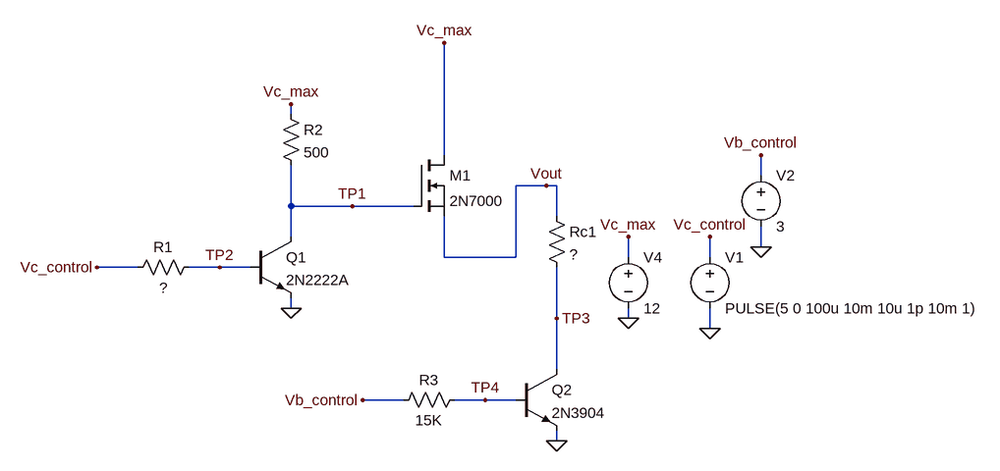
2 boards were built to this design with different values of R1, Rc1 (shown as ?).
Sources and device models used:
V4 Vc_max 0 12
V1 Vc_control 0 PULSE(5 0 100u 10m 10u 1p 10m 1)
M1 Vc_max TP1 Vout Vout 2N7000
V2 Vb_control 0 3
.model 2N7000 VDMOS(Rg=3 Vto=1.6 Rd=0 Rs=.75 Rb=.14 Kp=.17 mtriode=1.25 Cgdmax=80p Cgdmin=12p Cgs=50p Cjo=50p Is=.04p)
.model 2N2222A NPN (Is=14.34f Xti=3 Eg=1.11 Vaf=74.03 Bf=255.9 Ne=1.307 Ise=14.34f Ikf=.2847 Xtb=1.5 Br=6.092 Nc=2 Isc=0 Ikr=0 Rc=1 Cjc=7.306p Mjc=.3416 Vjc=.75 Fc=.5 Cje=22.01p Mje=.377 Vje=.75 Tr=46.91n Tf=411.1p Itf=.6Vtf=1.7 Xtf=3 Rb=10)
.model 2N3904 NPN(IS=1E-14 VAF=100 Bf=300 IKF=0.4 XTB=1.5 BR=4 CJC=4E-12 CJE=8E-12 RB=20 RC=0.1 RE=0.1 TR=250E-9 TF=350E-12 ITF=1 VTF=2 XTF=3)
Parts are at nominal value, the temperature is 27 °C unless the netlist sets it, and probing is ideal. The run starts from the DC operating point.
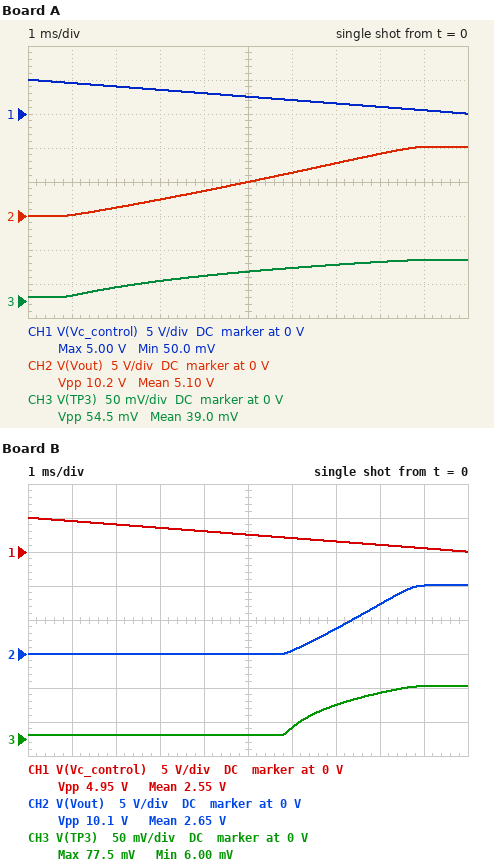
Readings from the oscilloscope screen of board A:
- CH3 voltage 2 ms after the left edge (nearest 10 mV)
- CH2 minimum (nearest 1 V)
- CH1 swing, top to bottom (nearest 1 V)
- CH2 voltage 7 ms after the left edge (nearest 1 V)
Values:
20 mV
0 V
5 V
8 V
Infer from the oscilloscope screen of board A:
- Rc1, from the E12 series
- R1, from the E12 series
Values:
2.2 kΩ
33 kΩ
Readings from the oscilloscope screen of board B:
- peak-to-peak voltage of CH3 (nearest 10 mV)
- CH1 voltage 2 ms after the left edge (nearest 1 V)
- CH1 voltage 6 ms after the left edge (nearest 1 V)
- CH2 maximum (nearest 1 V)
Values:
70 mV
4 V
2 V
10 V
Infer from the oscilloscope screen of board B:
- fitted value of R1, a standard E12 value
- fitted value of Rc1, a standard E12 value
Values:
12 kΩ
1.2 kΩ
